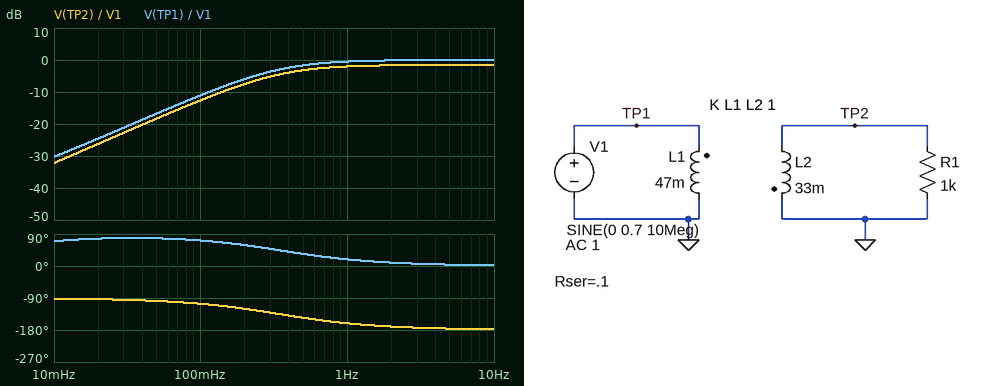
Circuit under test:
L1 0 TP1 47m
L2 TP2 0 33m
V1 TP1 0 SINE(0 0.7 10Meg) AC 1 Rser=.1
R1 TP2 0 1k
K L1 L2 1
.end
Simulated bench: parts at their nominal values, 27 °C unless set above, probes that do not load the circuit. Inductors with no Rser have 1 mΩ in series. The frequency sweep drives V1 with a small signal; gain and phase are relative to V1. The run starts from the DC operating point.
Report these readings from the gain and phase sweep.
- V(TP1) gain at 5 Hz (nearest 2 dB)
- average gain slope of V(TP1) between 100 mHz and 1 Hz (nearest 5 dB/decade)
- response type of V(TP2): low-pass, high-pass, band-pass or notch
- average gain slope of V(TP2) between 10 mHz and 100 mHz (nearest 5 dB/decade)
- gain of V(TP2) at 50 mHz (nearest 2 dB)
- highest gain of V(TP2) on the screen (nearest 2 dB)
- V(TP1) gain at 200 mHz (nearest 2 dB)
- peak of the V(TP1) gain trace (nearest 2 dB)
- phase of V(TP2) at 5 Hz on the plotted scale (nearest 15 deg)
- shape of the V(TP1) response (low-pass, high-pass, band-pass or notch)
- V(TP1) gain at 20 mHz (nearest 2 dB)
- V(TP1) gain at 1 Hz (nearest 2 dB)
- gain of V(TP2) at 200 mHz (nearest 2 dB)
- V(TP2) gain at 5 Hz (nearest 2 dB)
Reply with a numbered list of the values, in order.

1. 0 dB
2. 10 dB/decade
3. high-pass
4. 20 dB/decade
5. -18 dB
6. -2 dB
7. -6 dB
8. 0 dB
9. -180 deg
10. high-pass
11. -24 dB
12. 0 dB
13. -8 dB
14. -2 dB
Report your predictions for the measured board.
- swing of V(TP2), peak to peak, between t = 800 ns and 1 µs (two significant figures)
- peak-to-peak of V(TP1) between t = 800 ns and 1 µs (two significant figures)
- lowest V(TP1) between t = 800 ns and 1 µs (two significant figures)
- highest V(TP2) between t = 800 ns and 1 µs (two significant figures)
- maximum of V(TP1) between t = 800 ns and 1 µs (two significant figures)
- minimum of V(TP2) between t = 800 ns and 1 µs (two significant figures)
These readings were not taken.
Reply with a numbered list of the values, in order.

1. 1.2 V
2. 1.4 V
3. -700 mV
4. 590 mV
5. 700 mV
6. -590 mV
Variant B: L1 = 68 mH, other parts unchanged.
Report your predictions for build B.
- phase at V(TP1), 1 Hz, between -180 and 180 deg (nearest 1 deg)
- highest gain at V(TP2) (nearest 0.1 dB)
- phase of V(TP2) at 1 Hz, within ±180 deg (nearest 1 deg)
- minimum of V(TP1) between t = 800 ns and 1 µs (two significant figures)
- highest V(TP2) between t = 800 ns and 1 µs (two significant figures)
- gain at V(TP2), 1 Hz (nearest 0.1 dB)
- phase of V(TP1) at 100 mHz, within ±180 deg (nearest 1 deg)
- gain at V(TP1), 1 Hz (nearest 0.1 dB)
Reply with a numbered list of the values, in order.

1. 13 deg
2. -3.1 dB
3. -167 deg
4. -700 mV
5. 490 mV
6. -3.4 dB
7. 66 deg
8. -0.2 dB
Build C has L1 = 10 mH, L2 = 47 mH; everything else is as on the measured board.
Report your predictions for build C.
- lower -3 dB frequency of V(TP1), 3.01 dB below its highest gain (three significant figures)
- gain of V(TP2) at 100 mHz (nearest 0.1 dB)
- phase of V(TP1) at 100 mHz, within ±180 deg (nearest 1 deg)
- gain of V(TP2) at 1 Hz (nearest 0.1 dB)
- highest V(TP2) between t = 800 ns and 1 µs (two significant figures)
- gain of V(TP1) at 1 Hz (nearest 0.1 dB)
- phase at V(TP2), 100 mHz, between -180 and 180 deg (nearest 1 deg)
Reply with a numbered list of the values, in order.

1. 1.61 Hz
2. -17.4 dB
3. 77 deg
4. 1.2 dB
5. 1.5 V
6. -5.5 dB
7. -94 deg
